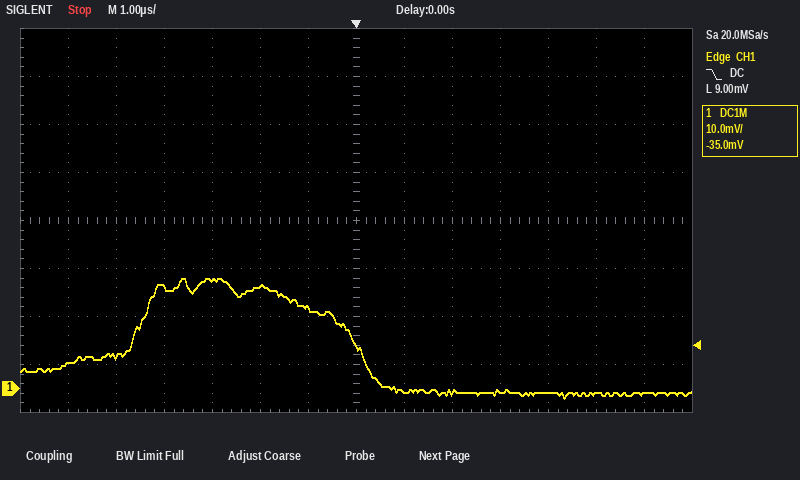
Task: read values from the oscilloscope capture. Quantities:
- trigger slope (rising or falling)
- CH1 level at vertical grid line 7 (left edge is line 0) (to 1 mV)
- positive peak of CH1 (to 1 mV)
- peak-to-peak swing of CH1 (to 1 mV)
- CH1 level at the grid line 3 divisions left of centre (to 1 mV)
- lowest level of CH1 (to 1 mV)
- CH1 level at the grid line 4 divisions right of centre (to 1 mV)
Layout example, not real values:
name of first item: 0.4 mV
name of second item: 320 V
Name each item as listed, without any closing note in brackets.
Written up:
trigger slope: falling
CH1 level at vertical grid line 7 (left edge is line 0): 9 mV
positive peak of CH1: 23 mV
peak-to-peak swing of CH1: 25 mV
CH1 level at the grid line 3 divisions left of centre: 23 mV
lowest level of CH1: -2 mV
CH1 level at the grid line 4 divisions right of centre: -1 mV
